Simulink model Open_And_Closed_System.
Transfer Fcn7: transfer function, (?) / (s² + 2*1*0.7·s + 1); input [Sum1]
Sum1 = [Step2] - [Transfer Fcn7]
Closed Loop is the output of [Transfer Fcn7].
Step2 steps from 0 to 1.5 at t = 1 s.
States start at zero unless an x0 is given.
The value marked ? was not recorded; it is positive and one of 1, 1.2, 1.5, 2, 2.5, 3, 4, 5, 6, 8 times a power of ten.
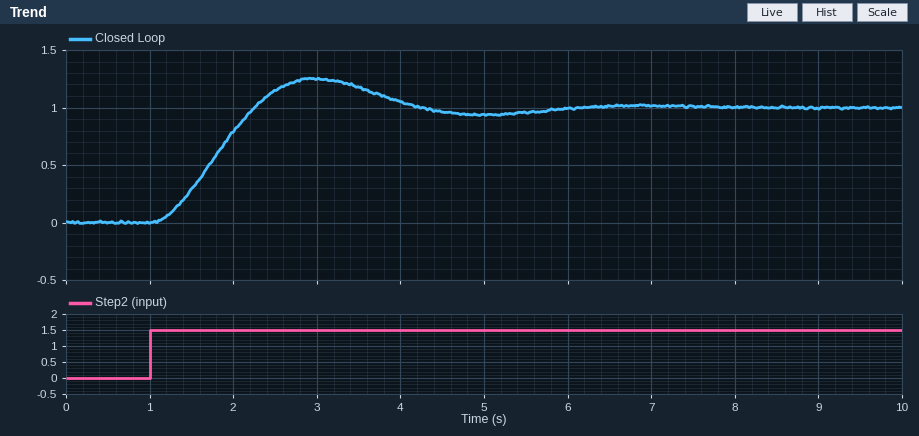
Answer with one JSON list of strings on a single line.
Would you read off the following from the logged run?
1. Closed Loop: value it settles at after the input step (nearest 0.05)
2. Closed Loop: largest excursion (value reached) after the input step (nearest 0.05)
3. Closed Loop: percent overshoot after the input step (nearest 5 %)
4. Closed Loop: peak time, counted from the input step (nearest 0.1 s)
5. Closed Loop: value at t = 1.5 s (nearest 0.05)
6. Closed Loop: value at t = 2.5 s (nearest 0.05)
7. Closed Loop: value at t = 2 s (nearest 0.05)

["1.00", "1.25", "25 %", "2.0 s", "0.30", "1.15", "0.80"]
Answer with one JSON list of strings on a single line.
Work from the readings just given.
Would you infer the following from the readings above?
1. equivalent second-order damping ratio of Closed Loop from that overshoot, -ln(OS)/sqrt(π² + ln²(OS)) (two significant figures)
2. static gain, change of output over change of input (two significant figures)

["0.40", "0.67"]
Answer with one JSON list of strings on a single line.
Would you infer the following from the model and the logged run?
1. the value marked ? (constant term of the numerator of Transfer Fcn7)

["2"]
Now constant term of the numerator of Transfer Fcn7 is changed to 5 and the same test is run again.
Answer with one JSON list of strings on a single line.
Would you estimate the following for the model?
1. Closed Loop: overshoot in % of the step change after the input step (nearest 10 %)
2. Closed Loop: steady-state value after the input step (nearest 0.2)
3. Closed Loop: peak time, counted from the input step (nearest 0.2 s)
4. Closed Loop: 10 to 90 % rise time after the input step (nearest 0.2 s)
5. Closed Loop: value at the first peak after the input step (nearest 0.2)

["40 %", "1.2", "1.4 s", "0.6 s", "1.8"]
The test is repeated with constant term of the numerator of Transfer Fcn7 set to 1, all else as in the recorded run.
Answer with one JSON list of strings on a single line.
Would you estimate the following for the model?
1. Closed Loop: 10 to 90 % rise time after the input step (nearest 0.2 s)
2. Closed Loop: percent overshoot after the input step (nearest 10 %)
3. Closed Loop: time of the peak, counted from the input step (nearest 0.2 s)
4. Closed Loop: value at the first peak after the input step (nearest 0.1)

["1.2 s", "20 %", "2.6 s", "0.9"]
